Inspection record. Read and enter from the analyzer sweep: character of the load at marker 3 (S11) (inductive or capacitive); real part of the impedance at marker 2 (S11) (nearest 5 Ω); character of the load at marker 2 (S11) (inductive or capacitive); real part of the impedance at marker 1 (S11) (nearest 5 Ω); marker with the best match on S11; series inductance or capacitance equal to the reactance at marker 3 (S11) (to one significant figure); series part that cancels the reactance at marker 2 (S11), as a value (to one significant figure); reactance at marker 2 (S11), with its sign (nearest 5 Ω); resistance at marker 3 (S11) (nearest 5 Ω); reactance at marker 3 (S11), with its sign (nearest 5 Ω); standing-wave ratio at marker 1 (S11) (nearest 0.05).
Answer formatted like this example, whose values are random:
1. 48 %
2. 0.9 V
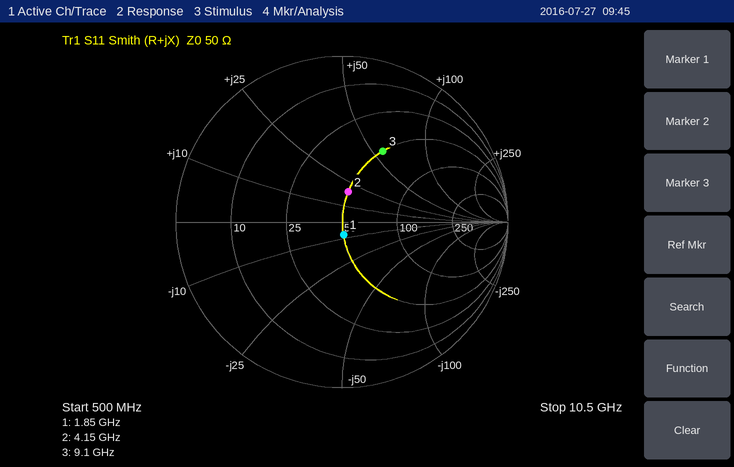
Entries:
1. inductive
2. 50 Ω
3. inductive
4. 50 Ω
5. marker 1
6. 1.0 nH
7. 2 pF
8. +20 Ω
9. 50 Ω
10. +55 Ω
11. 1.15
